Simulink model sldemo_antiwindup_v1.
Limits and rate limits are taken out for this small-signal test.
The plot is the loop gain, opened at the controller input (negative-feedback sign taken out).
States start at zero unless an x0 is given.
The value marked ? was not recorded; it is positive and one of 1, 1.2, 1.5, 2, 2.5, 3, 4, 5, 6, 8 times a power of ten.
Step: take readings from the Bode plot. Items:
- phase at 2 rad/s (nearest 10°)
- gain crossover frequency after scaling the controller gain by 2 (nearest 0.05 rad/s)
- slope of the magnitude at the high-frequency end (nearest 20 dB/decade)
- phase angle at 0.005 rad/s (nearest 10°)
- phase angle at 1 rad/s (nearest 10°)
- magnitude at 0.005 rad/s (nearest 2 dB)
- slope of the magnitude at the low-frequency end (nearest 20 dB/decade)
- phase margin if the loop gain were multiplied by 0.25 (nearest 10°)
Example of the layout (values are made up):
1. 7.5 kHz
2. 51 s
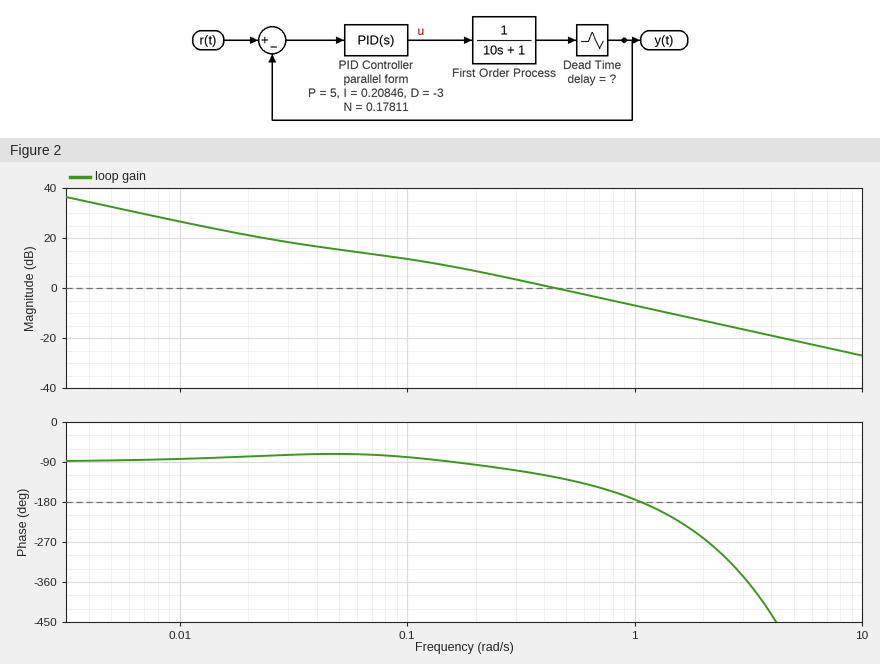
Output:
1. -260°
2. 0.90 rad/s
3. -20 dB/decade
4. -90°
5. -170°
6. 32 dB
7. -20 dB/decade
8. 100°
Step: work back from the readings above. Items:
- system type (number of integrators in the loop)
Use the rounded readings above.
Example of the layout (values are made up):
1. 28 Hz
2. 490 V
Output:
1. 1
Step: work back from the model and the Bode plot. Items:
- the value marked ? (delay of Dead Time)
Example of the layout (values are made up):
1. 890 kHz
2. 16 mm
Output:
1. 1.5
